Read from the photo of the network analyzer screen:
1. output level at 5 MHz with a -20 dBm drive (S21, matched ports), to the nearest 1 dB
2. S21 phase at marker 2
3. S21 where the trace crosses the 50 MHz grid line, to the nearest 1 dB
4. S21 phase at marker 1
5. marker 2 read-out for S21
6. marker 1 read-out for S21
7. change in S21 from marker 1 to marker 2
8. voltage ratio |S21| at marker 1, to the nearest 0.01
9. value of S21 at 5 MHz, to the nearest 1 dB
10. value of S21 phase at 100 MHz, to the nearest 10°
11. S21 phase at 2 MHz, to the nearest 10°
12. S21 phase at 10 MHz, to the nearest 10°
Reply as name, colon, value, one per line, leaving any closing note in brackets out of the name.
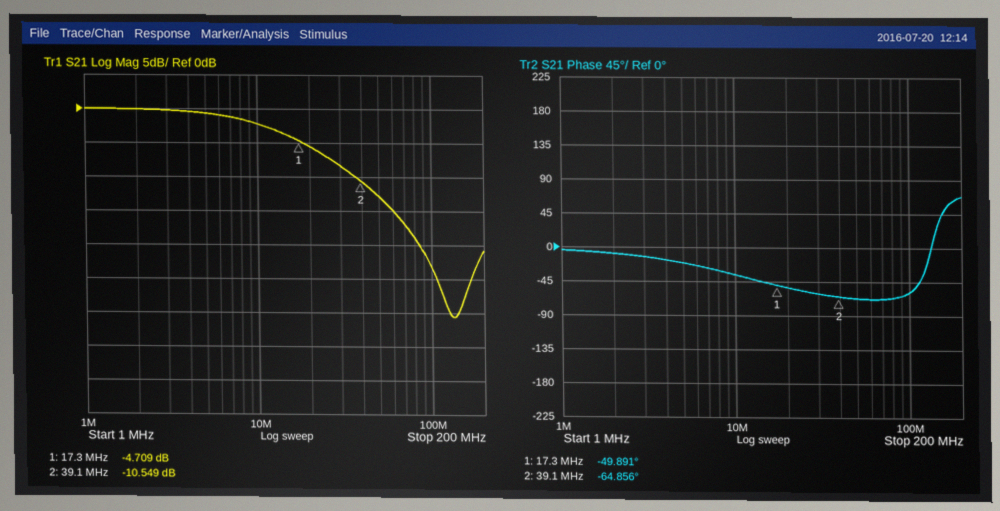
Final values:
output level at 5 MHz with a -20 dBm drive (S21, matched ports), to the nearest 1 dB: -21 dBm
S21 phase at marker 2: -64.856°
S21 where the trace crosses the 50 MHz grid line, to the nearest 1 dB: -13 dB
S21 phase at marker 1: -49.891°
marker 2 read-out for S21: -10.549 dB
marker 1 read-out for S21: -4.709 dB
change in S21 from marker 1 to marker 2: -5.840 dB
voltage ratio |S21| at marker 1, to the nearest 0.01: 0.58
value of S21 at 5 MHz, to the nearest 1 dB: -1 dB
value of S21 phase at 100 MHz, to the nearest 10°: -60°
S21 phase at 2 MHz, to the nearest 10°: -10°
S21 phase at 10 MHz, to the nearest 10°: -40°
